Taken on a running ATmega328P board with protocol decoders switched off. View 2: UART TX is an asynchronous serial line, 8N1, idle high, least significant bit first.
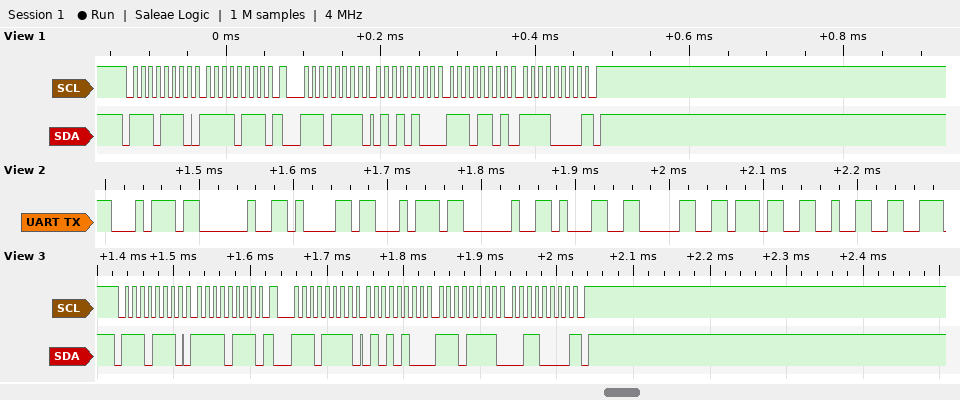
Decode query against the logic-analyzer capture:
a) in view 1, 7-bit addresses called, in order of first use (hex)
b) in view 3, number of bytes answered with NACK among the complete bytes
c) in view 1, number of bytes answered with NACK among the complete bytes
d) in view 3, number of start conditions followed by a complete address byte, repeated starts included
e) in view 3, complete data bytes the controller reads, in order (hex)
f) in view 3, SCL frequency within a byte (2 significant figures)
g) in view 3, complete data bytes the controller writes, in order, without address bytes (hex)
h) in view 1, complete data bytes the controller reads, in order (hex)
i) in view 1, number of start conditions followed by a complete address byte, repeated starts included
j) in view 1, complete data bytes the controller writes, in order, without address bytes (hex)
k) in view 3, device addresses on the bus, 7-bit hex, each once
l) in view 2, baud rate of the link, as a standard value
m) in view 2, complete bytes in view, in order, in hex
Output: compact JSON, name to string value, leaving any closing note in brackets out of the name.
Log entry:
{"in view 1, 7-bit addresses called, in order of first use": "0x77", "in view 3, number of bytes answered with NACK among the complete bytes": "1", "in view 1, number of bytes answered with NACK among the complete bytes": "1", "in view 3, number of start conditions followed by a complete address byte, repeated starts included": "2", "in view 3, complete data bytes the controller reads, in order": "54 EF 30", "in view 3, SCL frequency within a byte": "100 kHz", "in view 3, complete data bytes the controller writes, in order, without address bytes": "F7", "in view 1, complete data bytes the controller reads, in order": "54 ED F0", "in view 1, number of start conditions followed by a complete address byte, repeated starts included": "2", "in view 1, complete data bytes the controller writes, in order, without address bytes": "F7", "in view 3, device addresses on the bus, 7-bit hex, each once": "0x77", "in view 2, baud rate of the link, as a standard value": "115200 baud", "in view 2, complete bytes in view, in order, in hex": "74 20 61 74 20 31 30 37 32"}
